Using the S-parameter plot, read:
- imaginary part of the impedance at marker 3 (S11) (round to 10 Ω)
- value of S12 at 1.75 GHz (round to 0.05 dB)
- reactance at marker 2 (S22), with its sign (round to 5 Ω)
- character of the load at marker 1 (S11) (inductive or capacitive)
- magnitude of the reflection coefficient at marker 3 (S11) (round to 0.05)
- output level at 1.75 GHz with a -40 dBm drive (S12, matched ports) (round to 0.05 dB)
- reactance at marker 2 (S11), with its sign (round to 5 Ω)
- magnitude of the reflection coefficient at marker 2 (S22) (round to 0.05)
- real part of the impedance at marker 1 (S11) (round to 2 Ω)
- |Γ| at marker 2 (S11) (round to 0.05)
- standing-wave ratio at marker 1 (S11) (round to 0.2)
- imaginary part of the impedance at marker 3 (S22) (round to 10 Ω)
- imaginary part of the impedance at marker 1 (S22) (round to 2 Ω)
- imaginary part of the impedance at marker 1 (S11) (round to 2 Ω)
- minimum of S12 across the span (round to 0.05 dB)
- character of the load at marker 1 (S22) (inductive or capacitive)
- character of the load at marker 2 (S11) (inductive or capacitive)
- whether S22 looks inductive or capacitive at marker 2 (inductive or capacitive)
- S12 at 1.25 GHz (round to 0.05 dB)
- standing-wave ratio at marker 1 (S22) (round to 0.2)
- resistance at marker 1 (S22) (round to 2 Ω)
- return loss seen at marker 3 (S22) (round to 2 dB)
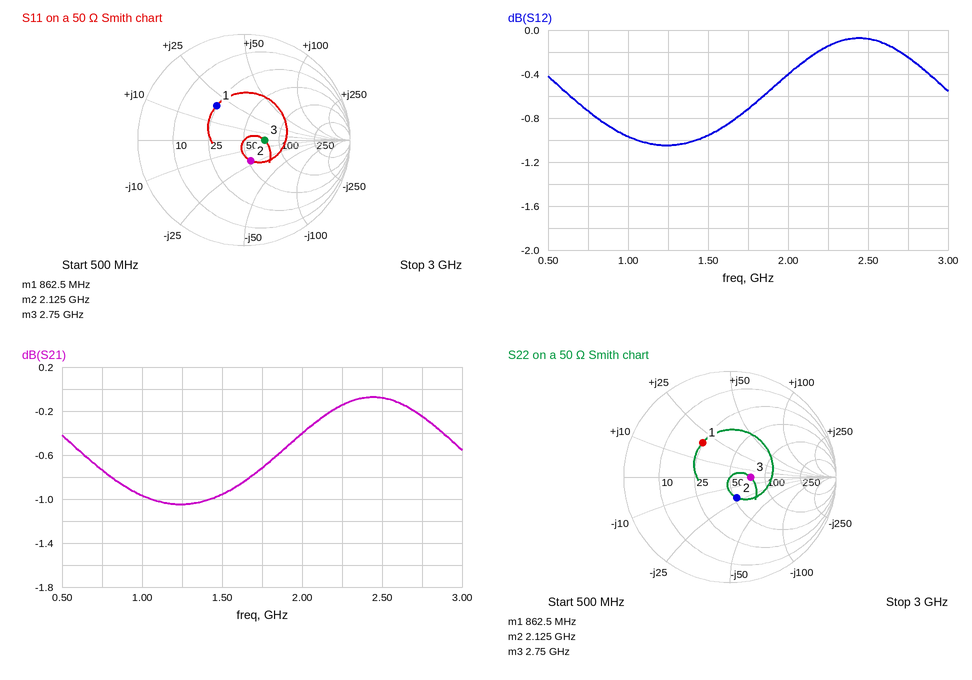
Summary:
0 Ω
-0.70 dB
-20 Ω
inductive
0.20
-40.70 dBm
-20 Ω
0.20
24 Ω
0.20
2.4
0 Ω
+20 Ω
+20 Ω
-1.05 dB
inductive
capacitive
capacitive
-1.05 dB
2.4
24 Ω
14 dB
